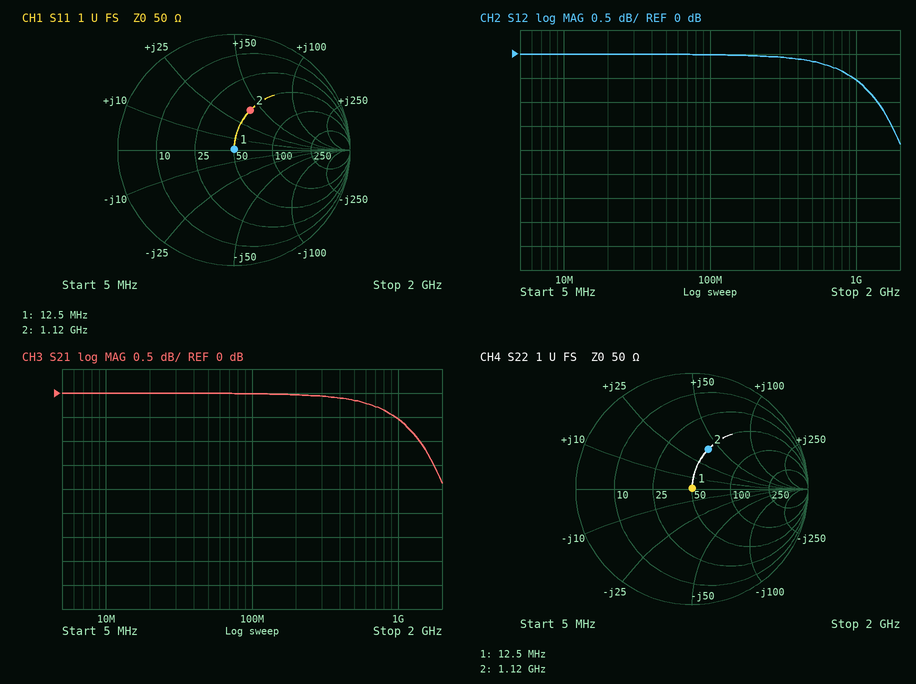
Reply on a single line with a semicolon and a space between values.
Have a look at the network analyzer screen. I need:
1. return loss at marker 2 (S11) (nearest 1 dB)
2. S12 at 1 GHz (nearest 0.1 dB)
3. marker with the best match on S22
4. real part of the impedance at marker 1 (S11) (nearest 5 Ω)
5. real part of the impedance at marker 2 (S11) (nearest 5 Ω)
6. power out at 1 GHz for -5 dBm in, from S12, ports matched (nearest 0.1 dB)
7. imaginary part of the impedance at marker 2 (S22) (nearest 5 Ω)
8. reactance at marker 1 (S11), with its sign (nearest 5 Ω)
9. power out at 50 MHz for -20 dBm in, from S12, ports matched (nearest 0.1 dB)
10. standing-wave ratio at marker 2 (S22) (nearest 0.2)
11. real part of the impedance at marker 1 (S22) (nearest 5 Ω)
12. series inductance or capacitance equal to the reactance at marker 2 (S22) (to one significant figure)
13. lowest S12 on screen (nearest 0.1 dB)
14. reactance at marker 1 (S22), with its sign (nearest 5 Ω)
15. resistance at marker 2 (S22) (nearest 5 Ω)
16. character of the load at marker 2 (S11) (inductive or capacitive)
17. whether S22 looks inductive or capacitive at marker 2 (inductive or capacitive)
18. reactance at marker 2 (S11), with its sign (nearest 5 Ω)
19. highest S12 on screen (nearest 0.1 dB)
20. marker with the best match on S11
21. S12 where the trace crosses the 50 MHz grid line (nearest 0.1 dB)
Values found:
9 dB; -0.5 dB; marker 1; 50 Ω; 50 Ω; -5.5 dBm; +40 Ω; 0 Ω; -20.0 dBm; 2.2; 50 Ω; 6 nH; -1.9 dB; 0 Ω; 50 Ω; inductive; inductive; +40 Ω; 0.0 dB; marker 1; 0.0 dB
